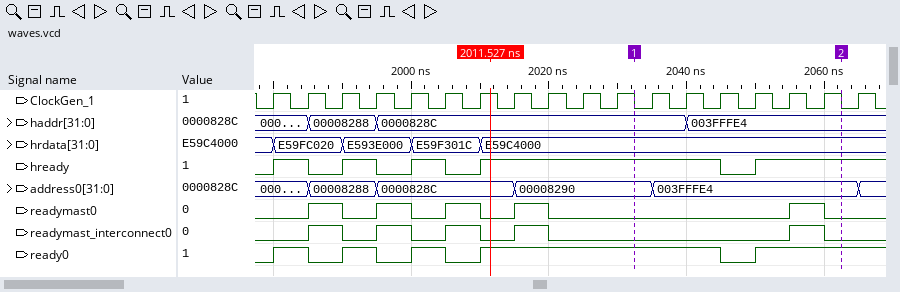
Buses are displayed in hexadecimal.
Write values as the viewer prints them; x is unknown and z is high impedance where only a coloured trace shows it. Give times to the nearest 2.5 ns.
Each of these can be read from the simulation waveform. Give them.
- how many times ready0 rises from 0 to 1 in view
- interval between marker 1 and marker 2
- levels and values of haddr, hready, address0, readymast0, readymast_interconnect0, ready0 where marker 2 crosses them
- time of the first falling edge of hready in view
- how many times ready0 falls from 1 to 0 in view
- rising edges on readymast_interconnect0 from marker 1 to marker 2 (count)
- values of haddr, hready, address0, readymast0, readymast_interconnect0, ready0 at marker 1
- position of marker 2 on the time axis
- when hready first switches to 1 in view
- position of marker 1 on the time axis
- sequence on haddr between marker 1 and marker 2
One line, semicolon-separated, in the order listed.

5; 30 ns; haddr=003FFFE4, hready=1, address0=003FFFE4, readymast0=0, readymast_interconnect0=0, ready0=1; 1985 ns; 4; 1; haddr=0000828C, hready=1, address0=00008290, readymast0=0, readymast_interconnect0=0, ready0=1; 2062.5 ns; 1980 ns; 2032.5 ns; 0000828C, 003FFFE4
